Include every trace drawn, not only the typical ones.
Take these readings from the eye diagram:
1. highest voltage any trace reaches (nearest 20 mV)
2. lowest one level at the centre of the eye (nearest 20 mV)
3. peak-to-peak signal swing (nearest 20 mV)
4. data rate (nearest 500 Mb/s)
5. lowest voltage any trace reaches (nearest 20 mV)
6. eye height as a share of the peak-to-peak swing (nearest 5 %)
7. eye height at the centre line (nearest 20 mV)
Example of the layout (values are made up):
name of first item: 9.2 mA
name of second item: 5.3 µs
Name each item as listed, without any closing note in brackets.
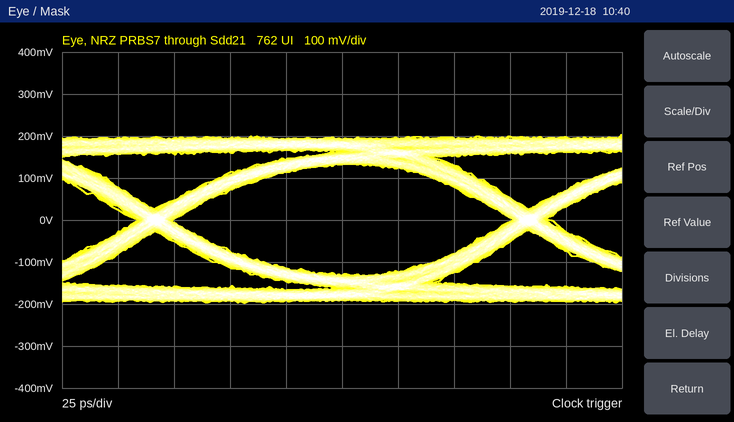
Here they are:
highest voltage any trace reaches: 200 mV
lowest one level at the centre of the eye: 140 mV
peak-to-peak signal swing: 400 mV
data rate: 6.0 Gb/s
lowest voltage any trace reaches: -200 mV
eye height as a share of the peak-to-peak swing: 65 %
eye height at the centre line: 260 mV
